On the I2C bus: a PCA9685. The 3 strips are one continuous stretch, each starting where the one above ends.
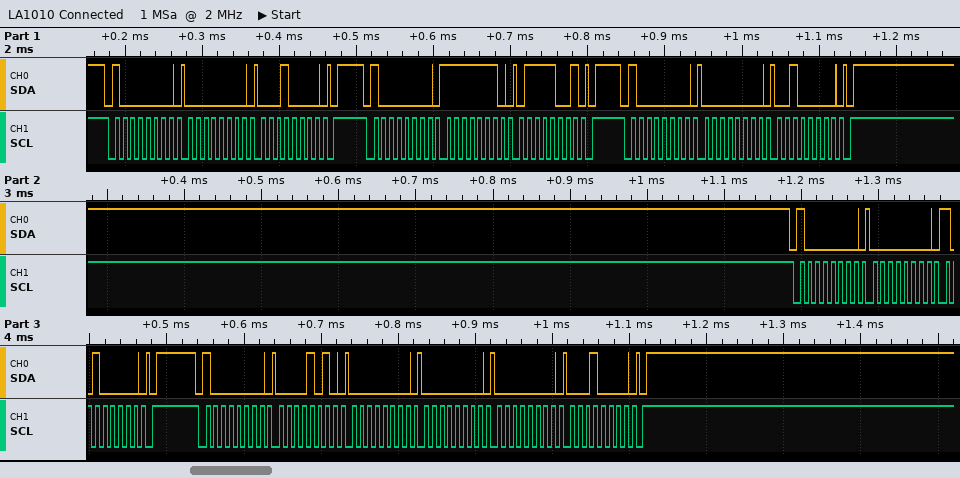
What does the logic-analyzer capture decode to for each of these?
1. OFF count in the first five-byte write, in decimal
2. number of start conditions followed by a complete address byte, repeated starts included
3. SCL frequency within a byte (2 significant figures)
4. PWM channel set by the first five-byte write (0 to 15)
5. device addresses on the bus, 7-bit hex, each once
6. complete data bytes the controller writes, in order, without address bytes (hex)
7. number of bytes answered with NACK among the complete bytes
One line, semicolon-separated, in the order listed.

4096; 5; 100 kHz; 1; 0x40; 00 10 FE 79 00 20 00 A0 0A 00 00 00 10; 0
